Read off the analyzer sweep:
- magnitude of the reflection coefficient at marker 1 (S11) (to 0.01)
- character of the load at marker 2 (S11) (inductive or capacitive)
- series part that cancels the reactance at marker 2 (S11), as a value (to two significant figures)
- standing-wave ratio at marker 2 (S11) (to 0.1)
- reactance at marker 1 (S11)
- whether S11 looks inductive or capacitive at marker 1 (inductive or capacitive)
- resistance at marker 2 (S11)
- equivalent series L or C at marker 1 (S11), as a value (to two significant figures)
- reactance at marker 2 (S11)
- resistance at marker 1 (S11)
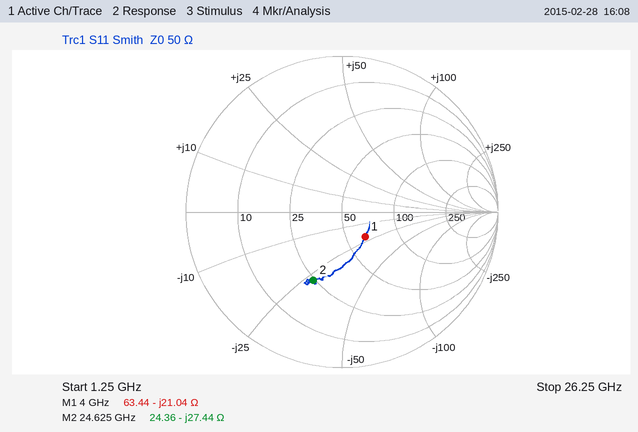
0.22
capacitive
180 pH
2.8
-21.04 Ω
capacitive
24.36 Ω
1.9 pF
-27.44 Ω
63.44 Ω
